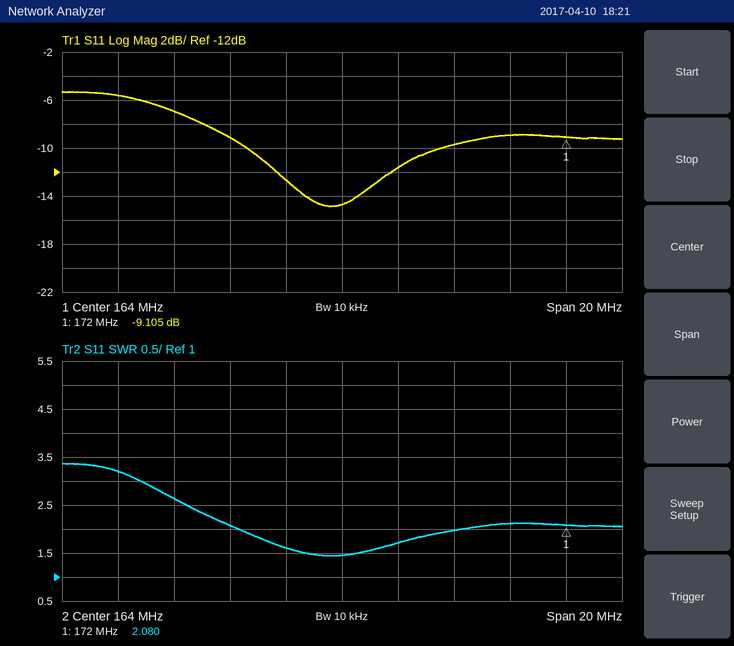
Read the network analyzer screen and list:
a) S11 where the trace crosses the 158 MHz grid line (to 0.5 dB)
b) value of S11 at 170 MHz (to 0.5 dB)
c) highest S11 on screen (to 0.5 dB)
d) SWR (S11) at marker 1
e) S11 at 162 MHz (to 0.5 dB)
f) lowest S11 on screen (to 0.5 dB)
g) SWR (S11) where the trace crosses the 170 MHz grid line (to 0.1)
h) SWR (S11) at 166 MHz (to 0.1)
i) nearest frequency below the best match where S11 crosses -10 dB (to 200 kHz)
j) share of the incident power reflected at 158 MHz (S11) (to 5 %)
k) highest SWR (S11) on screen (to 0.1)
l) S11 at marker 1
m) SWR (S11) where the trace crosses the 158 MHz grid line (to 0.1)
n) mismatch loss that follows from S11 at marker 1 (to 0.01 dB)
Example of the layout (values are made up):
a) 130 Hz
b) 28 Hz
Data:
a) -7.0 dB
b) -9.0 dB
c) -5.5 dB
d) 2.080
e) -12.5 dB
f) -15.0 dB
g) 2.1
h) 1.7
i) 160.6 MHz
j) 20 %
k) 3.4
l) -9.105 dB
m) 2.6
n) 0.57 dB
